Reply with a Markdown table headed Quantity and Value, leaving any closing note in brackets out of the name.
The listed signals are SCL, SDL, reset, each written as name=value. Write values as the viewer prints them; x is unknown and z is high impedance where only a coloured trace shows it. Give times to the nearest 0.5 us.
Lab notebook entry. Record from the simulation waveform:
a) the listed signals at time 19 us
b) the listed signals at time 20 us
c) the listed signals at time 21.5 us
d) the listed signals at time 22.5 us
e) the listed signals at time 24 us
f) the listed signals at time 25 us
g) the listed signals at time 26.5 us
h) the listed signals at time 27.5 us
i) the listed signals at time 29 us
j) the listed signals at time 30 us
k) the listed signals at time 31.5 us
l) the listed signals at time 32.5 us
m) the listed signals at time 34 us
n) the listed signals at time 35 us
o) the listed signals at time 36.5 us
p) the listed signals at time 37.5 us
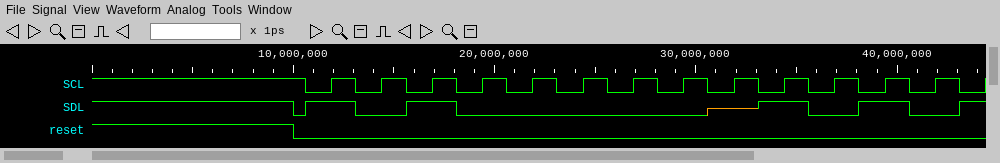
| Quantity | Value |
|---|---|
| the listed signals at time 19 us | SCL=0, SDL=0, reset=0 |
| the listed signals at time 20 us | SCL=1, SDL=0, reset=0 |
| the listed signals at time 21.5 us | SCL=0, SDL=0, reset=0 |
| the listed signals at time 22.5 us | SCL=1, SDL=0, reset=0 |
| the listed signals at time 24 us | SCL=0, SDL=0, reset=0 |
| the listed signals at time 25 us | SCL=1, SDL=0, reset=0 |
| the listed signals at time 26.5 us | SCL=0, SDL=0, reset=0 |
| the listed signals at time 27.5 us | SCL=1, SDL=0, reset=0 |
| the listed signals at time 29 us | SCL=0, SDL=0, reset=0 |
| the listed signals at time 30 us | SCL=1, SDL=0, reset=0 |
| the listed signals at time 31.5 us | SCL=0, SDL=z, reset=0 |
| the listed signals at time 32.5 us | SCL=1, SDL=z, reset=0 |
| the listed signals at time 34 us | SCL=0, SDL=1, reset=0 |
| the listed signals at time 35 us | SCL=1, SDL=1, reset=0 |
| the listed signals at time 36.5 us | SCL=0, SDL=0, reset=0 |
| the listed signals at time 37.5 us | SCL=1, SDL=0, reset=0 |
